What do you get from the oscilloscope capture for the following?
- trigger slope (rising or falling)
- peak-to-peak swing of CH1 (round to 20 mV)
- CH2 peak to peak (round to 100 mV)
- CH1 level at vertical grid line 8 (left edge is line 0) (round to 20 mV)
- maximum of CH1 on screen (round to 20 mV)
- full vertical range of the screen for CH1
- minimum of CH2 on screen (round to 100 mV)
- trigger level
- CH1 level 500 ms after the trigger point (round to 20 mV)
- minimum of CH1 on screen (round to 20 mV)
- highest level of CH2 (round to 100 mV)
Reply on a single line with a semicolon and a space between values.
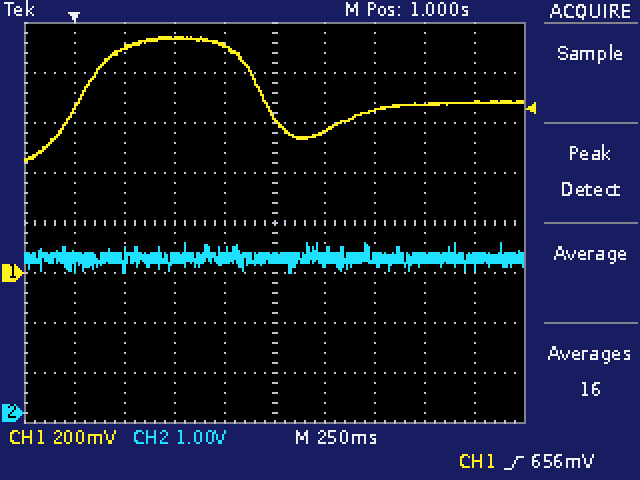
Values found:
rising; 500 mV; 600 mV; 680 mV; 940 mV; 1.6 V; 2.8 V; 656 mV; 940 mV; 440 mV; 3.4 V
